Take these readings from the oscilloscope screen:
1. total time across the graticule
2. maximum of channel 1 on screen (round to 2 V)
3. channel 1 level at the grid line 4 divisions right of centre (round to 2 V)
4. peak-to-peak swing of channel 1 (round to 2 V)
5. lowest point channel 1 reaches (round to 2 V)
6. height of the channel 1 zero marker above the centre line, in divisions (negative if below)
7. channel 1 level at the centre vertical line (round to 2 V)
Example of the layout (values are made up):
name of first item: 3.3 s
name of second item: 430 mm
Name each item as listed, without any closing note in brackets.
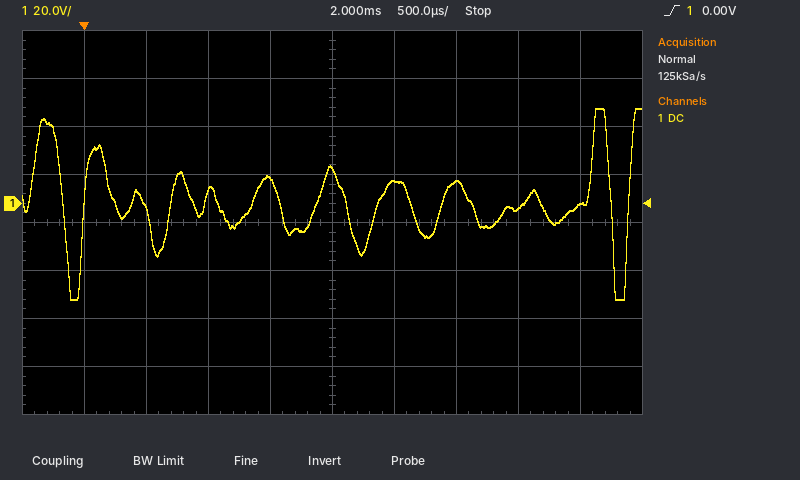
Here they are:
total time across the graticule: 5 ms
maximum of channel 1 on screen: 40 V
channel 1 level at the grid line 4 divisions right of centre: 0 V
peak-to-peak swing of channel 1: 80 V
lowest point channel 1 reaches: -40 V
height of the channel 1 zero marker above the centre line, in divisions: +0.4 div
channel 1 level at the centre vertical line: 14 V
